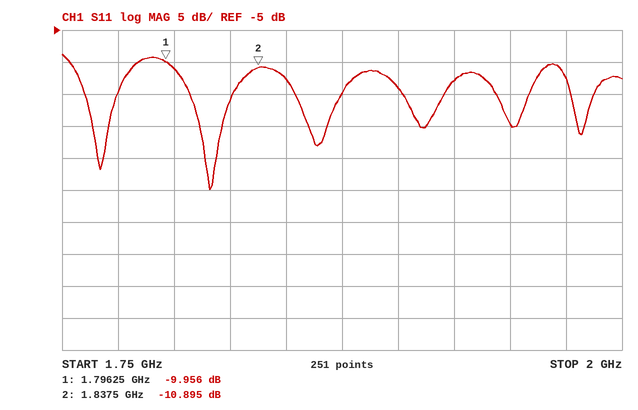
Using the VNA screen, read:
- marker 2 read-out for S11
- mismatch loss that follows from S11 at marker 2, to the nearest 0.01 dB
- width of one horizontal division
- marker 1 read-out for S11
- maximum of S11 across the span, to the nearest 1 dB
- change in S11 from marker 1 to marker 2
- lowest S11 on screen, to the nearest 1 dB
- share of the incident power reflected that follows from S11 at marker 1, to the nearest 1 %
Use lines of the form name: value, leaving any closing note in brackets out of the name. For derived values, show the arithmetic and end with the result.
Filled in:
marker 2 read-out for S11: -10.895 dB
mismatch loss that follows from S11 at marker 2, to the nearest 0.01 dB: −10 log10(1 − 10^(-10.895/10)) ≈ 0.37 dB
width of one horizontal division: 25 MHz
marker 1 read-out for S11: -9.956 dB
maximum of S11 across the span, to the nearest 1 dB: -9 dB
change in S11 from marker 1 to marker 2: -10.895 − (-9.956) = -0.939 dB
lowest S11 on screen, to the nearest 1 dB: -30 dB
share of the incident power reflected that follows from S11 at marker 1, to the nearest 1 %: 10^(-9.956/10) ≈ 10 %
